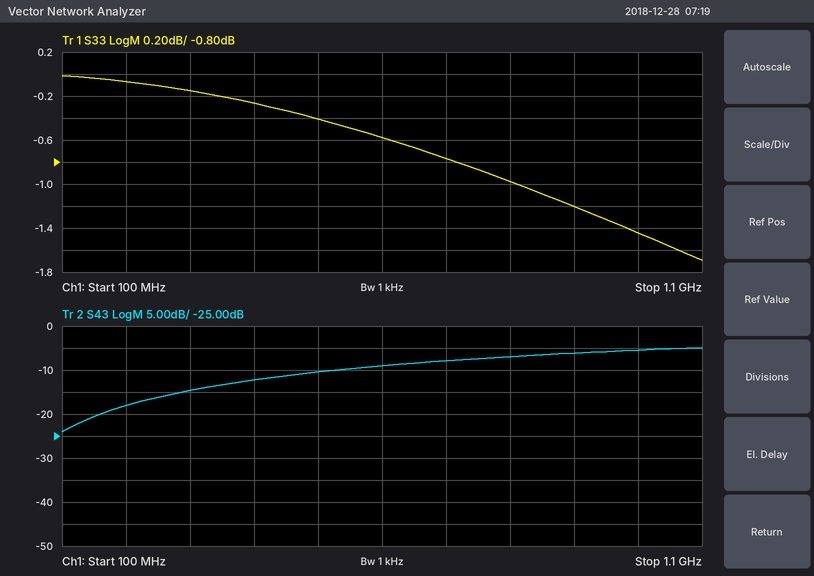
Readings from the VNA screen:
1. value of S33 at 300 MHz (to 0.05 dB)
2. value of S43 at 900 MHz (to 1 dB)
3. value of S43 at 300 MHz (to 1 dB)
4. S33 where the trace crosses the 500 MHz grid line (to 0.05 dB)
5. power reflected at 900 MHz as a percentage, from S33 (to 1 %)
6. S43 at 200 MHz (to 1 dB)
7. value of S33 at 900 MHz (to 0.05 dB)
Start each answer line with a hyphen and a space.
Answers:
- -0.15 dB
- -6 dB
- -15 dB
- -0.40 dB
- 76 %
- -18 dB
- -1.20 dB
